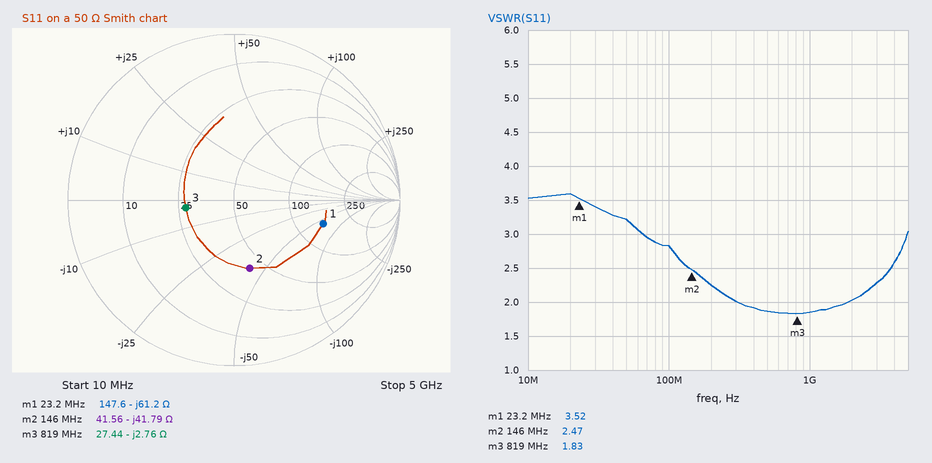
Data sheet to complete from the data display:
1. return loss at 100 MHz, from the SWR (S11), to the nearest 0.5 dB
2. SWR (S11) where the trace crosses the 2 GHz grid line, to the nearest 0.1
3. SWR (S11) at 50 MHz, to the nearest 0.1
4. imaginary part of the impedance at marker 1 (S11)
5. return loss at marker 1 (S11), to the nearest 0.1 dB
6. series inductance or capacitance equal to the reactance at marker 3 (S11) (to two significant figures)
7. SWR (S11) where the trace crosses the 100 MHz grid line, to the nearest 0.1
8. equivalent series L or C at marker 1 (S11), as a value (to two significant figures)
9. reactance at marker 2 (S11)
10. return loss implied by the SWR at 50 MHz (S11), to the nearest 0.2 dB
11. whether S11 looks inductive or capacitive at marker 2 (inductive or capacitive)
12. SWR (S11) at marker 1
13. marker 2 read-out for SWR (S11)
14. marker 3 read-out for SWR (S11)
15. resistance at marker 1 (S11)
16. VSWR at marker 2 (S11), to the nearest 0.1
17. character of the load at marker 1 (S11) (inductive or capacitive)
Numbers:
6.5 dB
2.0
3.2
-61.2 Ω
5.1 dB
70 pF
2.8
110 pF
-41.79 Ω
5.6 dB
capacitive
3.52
2.47
1.83
147.6 Ω
2.5
capacitive
